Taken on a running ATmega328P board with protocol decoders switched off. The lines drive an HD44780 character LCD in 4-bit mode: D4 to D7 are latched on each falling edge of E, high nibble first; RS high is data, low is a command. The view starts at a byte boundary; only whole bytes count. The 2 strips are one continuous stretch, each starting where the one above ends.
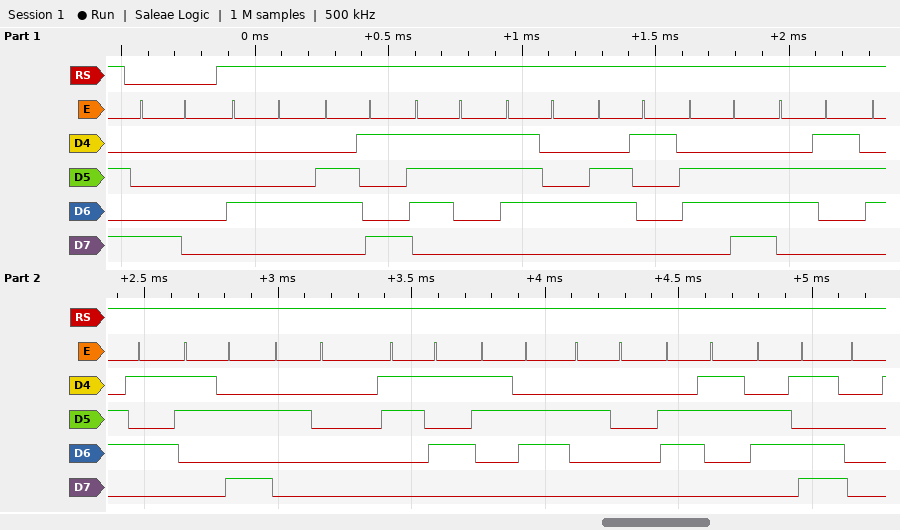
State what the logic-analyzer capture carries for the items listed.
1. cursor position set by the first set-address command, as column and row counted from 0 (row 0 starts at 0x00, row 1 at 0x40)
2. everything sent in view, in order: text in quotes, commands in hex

column 0, row 0
0x80 "Distance: 56 cm"
